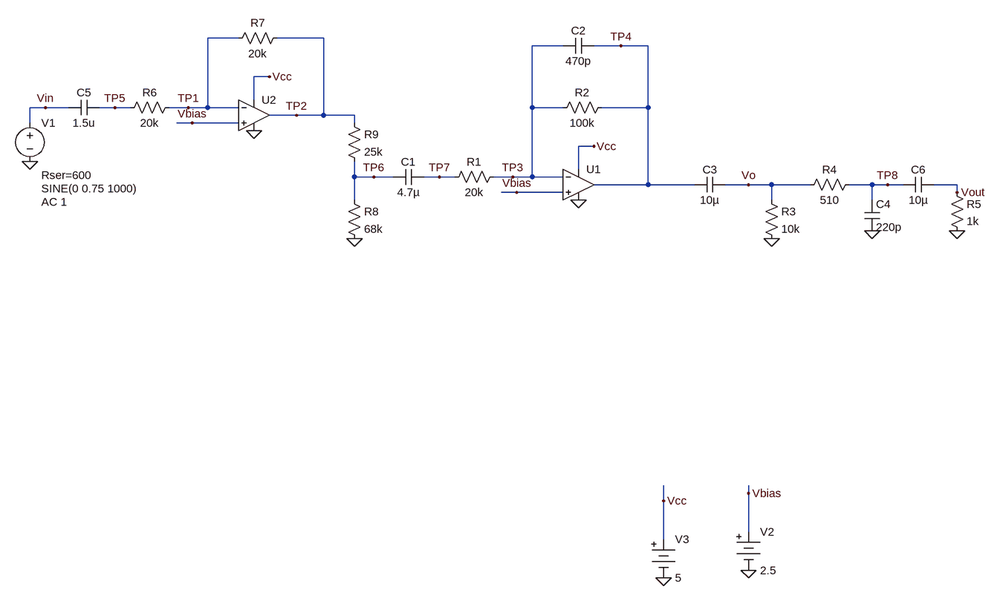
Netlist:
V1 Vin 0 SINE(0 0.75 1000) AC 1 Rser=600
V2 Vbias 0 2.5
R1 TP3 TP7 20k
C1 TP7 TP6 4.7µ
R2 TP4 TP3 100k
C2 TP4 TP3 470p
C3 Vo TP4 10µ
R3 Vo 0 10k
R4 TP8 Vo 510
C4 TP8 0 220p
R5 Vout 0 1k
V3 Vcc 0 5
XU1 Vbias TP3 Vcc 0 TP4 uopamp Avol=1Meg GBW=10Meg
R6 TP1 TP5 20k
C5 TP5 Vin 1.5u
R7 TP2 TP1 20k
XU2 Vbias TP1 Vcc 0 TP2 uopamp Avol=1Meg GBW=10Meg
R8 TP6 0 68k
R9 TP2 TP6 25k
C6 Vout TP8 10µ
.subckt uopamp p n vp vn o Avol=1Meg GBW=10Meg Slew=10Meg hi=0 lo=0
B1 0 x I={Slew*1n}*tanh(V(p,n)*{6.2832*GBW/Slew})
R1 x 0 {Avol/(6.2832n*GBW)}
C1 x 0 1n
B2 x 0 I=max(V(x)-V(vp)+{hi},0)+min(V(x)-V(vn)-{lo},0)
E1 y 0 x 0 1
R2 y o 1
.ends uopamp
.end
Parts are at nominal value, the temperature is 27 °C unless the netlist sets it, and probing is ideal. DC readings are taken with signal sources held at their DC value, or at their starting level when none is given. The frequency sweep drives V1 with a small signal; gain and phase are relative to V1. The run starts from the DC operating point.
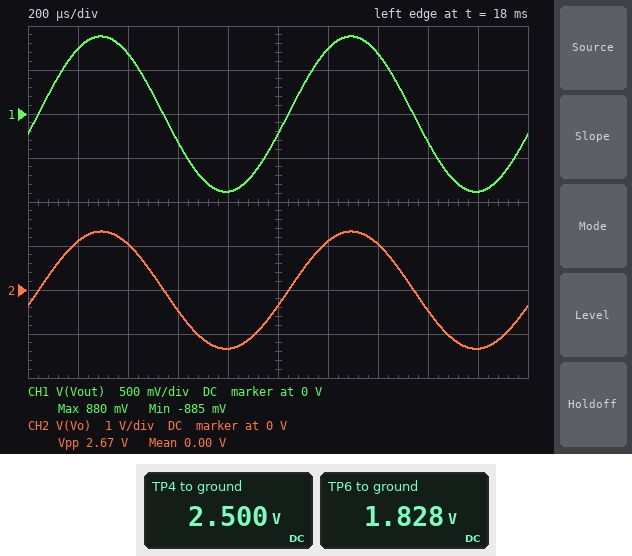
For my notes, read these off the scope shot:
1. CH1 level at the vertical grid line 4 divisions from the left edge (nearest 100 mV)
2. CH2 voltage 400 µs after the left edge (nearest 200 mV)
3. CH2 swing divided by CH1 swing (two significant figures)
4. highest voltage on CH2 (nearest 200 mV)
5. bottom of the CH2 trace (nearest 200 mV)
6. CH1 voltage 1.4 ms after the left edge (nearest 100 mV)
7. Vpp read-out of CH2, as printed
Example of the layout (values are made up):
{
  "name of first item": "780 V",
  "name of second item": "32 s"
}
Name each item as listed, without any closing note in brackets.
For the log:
{
  "CH1 level at the vertical grid line 4 divisions from the left edge": "-900 mV",
  "CH2 voltage 400 µs after the left edge": "1.0 V",
  "CH2 swing divided by CH1 swing": "1.5",
  "highest voltage on CH2": "1.4 V",
  "bottom of the CH2 trace": "-1.4 V",
  "CH1 voltage 1.4 ms after the left edge": "700 mV",
  "Vpp read-out of CH2, as printed": "2.67 V"
}
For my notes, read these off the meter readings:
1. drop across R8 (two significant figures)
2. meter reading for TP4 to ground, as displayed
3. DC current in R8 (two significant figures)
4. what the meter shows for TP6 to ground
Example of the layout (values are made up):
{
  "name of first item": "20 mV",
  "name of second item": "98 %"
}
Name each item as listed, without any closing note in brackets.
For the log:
{
  "drop across R8": "1.8 V",
  "meter reading for TP4 to ground, as displayed": "2.500 V",
  "DC current in R8": "27 µA",
  "what the meter shows for TP6 to ground": "1.828 V"
}
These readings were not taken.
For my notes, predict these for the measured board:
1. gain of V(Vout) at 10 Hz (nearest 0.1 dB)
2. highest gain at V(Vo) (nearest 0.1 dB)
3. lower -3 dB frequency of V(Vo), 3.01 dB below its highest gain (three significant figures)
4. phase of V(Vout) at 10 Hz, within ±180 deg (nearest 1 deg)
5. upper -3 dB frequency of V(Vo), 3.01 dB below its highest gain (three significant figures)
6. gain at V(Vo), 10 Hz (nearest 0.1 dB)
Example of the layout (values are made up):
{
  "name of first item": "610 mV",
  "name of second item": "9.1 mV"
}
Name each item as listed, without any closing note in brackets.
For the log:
{
  "gain of V(Vout) at 10 Hz": "-6.9 dB",
  "highest gain at V(Vo)": "5.3 dB",
  "lower -3 dB frequency of V(Vo), 3.01 dB below its highest gain": "17.8 Hz",
  "phase of V(Vout) at 10 Hz, within ±180 deg": "102 deg",
  "upper -3 dB frequency of V(Vo), 3.01 dB below its highest gain": "3.42 kHz",
  "gain at V(Vo), 10 Hz": "-0.1 dB"
}
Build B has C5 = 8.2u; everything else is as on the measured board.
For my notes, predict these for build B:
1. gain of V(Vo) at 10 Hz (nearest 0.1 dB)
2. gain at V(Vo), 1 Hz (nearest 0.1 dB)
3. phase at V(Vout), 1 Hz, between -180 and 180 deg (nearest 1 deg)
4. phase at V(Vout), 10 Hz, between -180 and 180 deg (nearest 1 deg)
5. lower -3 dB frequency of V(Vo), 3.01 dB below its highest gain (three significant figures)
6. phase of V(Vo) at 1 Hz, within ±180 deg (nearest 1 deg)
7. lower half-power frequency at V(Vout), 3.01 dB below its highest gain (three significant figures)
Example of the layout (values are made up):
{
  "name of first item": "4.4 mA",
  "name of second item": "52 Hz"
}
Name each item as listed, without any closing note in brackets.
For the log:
{
  "gain of V(Vo) at 10 Hz": "0.9 dB",
  "gain at V(Vo), 1 Hz": "-8.2 dB",
  "phase at V(Vout), 1 Hz, between -180 and 180 deg": "-150 deg",
  "phase at V(Vout), 10 Hz, between -180 and 180 deg": "80 deg",
  "lower -3 dB frequency of V(Vo), 3.01 dB below its highest gain": "16.0 Hz",
  "phase of V(Vo) at 1 Hz, within ±180 deg": "125 deg",
  "lower half-power frequency at V(Vout), 3.01 dB below its highest gain": "21.7 Hz"
}
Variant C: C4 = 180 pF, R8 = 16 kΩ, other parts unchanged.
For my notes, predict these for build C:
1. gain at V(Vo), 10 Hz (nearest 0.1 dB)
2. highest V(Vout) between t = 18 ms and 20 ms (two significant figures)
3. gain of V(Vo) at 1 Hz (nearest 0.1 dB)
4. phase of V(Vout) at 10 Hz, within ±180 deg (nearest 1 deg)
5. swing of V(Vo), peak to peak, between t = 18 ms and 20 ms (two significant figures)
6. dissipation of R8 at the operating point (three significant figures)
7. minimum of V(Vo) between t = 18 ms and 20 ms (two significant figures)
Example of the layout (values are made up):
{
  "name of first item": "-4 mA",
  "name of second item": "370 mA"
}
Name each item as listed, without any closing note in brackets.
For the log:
{
  "gain at V(Vo), 10 Hz": "-3.4 dB",
  "highest V(Vout) between t = 18 ms and 20 ms": "610 mV",
  "gain of V(Vo) at 1 Hz": "-24.2 dB",
  "phase of V(Vout) at 10 Hz, within ±180 deg": "103 deg",
  "swing of V(Vo), peak to peak, between t = 18 ms and 20 ms": "1.8 V",
  "dissipation of R8 at the operating point": "59.5 µW",
  "minimum of V(Vo) between t = 18 ms and 20 ms": "-920 mV"
}
